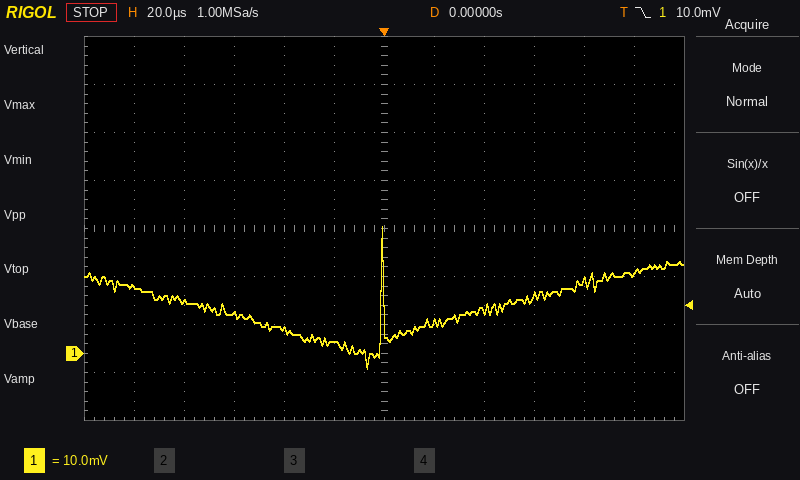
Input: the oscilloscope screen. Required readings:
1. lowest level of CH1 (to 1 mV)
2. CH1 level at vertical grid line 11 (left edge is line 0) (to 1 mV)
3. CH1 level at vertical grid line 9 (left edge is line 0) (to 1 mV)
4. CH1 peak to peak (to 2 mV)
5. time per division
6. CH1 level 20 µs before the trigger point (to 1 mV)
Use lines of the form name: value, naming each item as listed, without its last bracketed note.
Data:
lowest level of CH1: -3 mV
CH1 level at vertical grid line 11 (left edge is line 0): 17 mV
CH1 level at vertical grid line 9 (left edge is line 0): 12 mV
CH1 peak to peak: 30 mV
time per division: 20 µs
CH1 level 20 µs before the trigger point: 2 mV
